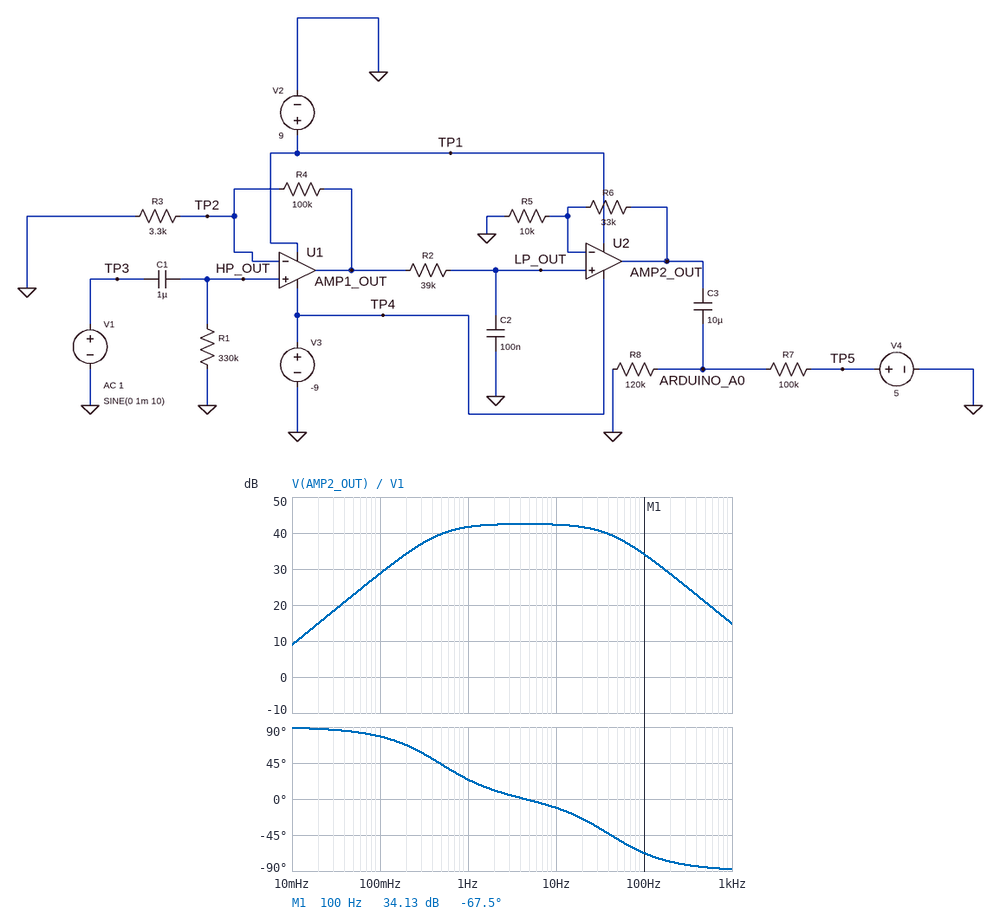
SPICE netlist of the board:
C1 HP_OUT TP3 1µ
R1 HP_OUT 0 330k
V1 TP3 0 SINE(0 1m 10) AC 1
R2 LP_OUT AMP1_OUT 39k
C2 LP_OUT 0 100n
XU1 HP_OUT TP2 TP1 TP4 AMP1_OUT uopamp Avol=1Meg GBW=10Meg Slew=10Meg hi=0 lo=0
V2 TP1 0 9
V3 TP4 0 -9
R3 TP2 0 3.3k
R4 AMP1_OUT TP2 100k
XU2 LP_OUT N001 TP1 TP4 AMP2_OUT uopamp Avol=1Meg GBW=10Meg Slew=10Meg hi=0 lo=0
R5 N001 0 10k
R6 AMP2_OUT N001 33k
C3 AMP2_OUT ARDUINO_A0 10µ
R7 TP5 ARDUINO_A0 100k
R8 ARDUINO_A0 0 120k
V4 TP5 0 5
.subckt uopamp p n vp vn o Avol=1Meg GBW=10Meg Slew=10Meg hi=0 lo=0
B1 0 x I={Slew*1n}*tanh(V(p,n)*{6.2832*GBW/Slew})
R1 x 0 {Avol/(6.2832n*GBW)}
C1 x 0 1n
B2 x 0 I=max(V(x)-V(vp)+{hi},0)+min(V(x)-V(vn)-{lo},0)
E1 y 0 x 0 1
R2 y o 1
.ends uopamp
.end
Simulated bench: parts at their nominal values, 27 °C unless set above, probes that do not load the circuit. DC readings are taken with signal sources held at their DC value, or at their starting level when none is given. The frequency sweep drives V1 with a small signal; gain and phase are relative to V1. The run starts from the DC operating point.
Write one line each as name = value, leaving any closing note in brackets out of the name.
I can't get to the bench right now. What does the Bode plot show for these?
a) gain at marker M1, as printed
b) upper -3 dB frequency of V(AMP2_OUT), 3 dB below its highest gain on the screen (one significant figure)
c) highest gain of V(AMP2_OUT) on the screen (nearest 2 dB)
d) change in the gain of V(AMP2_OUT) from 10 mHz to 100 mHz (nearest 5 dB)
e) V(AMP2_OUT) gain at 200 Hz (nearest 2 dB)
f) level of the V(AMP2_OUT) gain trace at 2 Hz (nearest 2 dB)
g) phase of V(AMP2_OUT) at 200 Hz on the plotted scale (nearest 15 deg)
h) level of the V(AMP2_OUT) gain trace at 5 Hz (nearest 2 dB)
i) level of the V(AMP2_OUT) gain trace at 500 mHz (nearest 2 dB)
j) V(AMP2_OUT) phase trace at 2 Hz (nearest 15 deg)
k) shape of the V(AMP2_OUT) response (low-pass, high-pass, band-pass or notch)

gain at marker M1, as printed = 34.13 dB
upper -3 dB frequency of V(AMP2_OUT), 3 dB below its highest gain on the screen = 40 Hz
highest gain of V(AMP2_OUT) on the screen = 42 dB
change in the gain of V(AMP2_OUT) from 10 mHz to 100 mHz = 20 dB
V(AMP2_OUT) gain at 200 Hz = 28 dB
level of the V(AMP2_OUT) gain trace at 2 Hz = 42 dB
phase of V(AMP2_OUT) at 200 Hz on the plotted scale = -75 deg
level of the V(AMP2_OUT) gain trace at 5 Hz = 42 dB
level of the V(AMP2_OUT) gain trace at 500 mHz = 40 dB
V(AMP2_OUT) phase trace at 2 Hz = 15 deg
shape of the V(AMP2_OUT) response = band-pass
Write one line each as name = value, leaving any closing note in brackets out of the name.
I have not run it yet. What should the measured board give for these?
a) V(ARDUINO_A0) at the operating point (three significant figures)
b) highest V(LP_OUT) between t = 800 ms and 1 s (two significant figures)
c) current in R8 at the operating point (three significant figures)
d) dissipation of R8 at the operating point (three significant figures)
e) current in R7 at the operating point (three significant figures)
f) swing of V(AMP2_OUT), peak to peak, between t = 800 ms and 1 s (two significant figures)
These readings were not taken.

V(ARDUINO_A0) at the operating point = 2.73 V
highest V(LP_OUT) between t = 800 ms and 1 s = 30 mV
current in R8 at the operating point = 22.7 µA
dissipation of R8 at the operating point = 62.0 µW
current in R7 at the operating point = 22.7 µA
swing of V(AMP2_OUT), peak to peak, between t = 800 ms and 1 s = 260 mV
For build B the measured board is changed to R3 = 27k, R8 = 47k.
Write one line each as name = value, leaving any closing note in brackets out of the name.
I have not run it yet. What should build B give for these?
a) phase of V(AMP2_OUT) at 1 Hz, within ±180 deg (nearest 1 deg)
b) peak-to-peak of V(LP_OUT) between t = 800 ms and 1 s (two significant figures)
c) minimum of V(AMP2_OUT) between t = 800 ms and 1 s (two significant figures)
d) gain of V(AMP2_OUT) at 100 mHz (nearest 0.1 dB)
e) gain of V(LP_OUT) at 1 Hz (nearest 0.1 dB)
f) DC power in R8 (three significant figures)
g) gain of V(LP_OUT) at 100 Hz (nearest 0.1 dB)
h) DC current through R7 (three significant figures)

phase of V(AMP2_OUT) at 1 Hz, within ±180 deg = 24 deg
peak-to-peak of V(LP_OUT) between t = 800 ms and 1 s = 9.1 mV
minimum of V(AMP2_OUT) between t = 800 ms and 1 s = -20 mV
gain of V(AMP2_OUT) at 100 mHz = 12.3 dB
gain of V(LP_OUT) at 1 Hz = 12.5 dB
DC power in R8 = 54.4 µW
gain of V(LP_OUT) at 100 Hz = 5.0 dB
DC current through R7 = 34.0 µA
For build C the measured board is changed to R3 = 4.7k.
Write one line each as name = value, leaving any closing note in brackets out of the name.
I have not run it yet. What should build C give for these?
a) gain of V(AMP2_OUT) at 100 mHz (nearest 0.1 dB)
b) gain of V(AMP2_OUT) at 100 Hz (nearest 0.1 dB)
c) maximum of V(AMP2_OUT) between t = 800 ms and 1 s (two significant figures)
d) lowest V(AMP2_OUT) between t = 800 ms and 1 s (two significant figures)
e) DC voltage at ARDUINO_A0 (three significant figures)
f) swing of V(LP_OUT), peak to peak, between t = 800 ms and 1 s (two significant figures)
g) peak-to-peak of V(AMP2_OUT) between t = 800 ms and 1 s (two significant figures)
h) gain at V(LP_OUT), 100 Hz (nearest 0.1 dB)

gain of V(AMP2_OUT) at 100 mHz = 25.8 dB
gain of V(AMP2_OUT) at 100 Hz = 31.2 dB
maximum of V(AMP2_OUT) between t = 800 ms and 1 s = 93 mV
lowest V(AMP2_OUT) between t = 800 ms and 1 s = -93 mV
DC voltage at ARDUINO_A0 = 2.73 V
swing of V(LP_OUT), peak to peak, between t = 800 ms and 1 s = 43 mV
peak-to-peak of V(AMP2_OUT) between t = 800 ms and 1 s = 190 mV
gain at V(LP_OUT), 100 Hz = 18.5 dB
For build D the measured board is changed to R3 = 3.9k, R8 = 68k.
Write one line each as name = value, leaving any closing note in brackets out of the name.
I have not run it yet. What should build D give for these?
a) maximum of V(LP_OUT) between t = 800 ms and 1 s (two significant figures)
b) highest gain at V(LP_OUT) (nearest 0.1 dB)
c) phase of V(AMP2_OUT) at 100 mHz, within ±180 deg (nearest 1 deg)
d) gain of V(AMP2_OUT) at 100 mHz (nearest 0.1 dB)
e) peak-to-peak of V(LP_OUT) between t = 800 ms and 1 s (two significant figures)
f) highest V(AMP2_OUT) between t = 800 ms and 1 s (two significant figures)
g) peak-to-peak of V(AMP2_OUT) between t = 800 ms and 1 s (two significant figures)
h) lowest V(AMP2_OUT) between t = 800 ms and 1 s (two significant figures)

maximum of V(LP_OUT) between t = 800 ms and 1 s = 26 mV
highest gain at V(LP_OUT) = 28.4 dB
phase of V(AMP2_OUT) at 100 mHz, within ±180 deg = 78 deg
gain of V(AMP2_OUT) at 100 mHz = 27.3 dB
peak-to-peak of V(LP_OUT) between t = 800 ms and 1 s = 52 mV
highest V(AMP2_OUT) between t = 800 ms and 1 s = 110 mV
peak-to-peak of V(AMP2_OUT) between t = 800 ms and 1 s = 220 mV
lowest V(AMP2_OUT) between t = 800 ms and 1 s = -110 mV
